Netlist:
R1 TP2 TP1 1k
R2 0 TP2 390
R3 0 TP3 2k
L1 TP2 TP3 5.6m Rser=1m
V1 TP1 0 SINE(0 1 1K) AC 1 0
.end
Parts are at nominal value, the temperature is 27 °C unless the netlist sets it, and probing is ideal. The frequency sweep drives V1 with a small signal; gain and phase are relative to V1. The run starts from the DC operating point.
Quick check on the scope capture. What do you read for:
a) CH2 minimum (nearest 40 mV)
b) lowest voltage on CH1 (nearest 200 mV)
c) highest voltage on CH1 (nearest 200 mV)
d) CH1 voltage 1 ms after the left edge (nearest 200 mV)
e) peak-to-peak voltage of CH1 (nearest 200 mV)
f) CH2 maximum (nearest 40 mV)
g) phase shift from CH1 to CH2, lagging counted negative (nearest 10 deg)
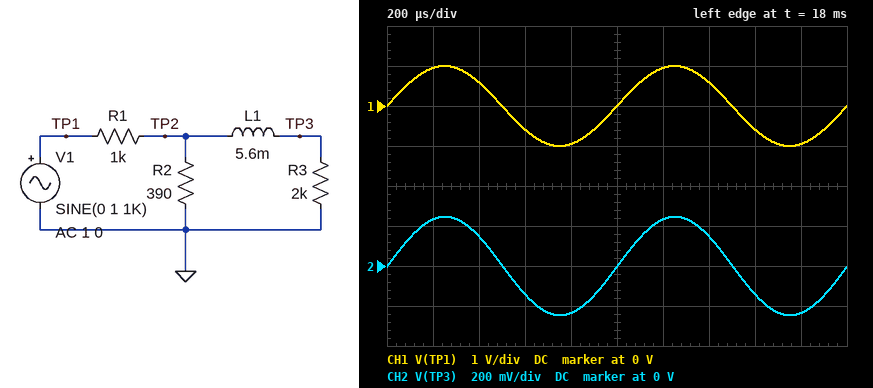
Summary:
-240 mV
-1.0 V
1.0 V
0 V
2.0 V
240 mV
0 deg
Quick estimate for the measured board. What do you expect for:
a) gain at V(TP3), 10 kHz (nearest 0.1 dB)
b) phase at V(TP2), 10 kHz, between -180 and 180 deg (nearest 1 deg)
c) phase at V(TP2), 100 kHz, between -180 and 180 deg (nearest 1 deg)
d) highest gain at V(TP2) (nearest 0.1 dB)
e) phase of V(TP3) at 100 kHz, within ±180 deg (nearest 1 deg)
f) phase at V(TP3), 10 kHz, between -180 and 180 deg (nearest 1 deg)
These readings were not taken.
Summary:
-12.3 dB
1 deg
3 deg
-11.0 dB
-57 deg
-9 deg
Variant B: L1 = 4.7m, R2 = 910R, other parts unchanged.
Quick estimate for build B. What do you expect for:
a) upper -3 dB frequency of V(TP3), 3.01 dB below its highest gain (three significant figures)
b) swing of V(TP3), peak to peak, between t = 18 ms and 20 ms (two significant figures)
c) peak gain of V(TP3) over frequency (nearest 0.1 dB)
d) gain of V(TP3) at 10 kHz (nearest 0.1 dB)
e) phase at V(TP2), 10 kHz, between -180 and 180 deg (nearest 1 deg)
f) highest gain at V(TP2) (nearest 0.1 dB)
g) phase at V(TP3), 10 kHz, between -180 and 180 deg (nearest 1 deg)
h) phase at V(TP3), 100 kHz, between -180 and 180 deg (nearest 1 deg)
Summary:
83.9 kHz
770 mV
-8.3 dB
-8.4 dB
2 deg
-6.4 dB
-7 deg
-50 deg
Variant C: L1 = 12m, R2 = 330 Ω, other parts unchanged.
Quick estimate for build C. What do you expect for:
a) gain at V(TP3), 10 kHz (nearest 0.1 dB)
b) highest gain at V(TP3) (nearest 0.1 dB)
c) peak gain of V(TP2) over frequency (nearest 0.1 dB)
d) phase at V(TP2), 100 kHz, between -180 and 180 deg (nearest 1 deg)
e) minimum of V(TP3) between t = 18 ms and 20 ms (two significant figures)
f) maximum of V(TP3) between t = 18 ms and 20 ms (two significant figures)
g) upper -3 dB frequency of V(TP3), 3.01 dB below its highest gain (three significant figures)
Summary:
-13.6 dB
-13.1 dB
-12.1 dB
2 deg
-220 mV
220 mV
29.8 kHz
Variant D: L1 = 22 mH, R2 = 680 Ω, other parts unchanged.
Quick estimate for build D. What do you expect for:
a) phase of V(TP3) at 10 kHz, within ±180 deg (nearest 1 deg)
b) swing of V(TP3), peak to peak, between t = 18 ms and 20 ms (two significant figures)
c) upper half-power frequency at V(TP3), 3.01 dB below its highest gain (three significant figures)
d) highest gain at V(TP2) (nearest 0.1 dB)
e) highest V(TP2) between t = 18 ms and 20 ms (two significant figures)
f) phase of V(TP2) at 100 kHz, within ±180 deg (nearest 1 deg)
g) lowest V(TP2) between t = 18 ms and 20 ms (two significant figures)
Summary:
-30 deg
670 mV
17.4 kHz
-7.9 dB
340 mV
2 deg
-340 mV
